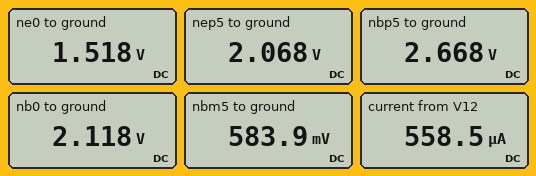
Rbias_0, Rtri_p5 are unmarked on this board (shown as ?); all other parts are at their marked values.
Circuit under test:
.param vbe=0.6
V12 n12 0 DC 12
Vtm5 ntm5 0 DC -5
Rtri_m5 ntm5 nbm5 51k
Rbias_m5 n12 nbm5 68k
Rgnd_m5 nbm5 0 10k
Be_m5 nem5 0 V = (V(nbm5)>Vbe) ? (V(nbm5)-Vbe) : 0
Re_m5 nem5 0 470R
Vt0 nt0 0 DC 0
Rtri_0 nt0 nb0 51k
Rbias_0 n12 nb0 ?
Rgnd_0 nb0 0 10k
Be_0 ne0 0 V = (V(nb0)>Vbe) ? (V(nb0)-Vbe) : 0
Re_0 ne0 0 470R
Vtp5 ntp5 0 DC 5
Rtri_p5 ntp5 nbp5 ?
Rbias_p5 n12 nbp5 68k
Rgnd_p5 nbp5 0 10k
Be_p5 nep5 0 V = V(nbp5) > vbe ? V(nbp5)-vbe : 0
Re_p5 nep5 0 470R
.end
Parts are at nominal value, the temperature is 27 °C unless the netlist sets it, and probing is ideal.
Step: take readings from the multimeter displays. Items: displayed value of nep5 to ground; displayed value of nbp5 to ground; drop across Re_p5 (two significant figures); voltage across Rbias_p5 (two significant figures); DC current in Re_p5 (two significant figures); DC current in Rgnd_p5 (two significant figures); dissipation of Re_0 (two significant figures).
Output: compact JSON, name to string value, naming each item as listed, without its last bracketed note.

{"displayed value of nep5 to ground": "2.068 V", "displayed value of nbp5 to ground": "2.668 V", "drop across Re_p5": "2.1 V", "voltage across Rbias_p5": "9.3 V", "DC current in Re_p5": "4.4 mA", "DC current in Rgnd_p5": "270 µA", "dissipation of Re_0": "4.9 mW"}
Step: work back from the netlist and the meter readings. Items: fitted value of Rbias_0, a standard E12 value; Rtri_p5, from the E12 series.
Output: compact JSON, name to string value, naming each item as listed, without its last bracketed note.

{"fitted value of Rbias_0, a standard E12 value": "39 kΩ", "Rtri_p5, from the E12 series": "18 kΩ"}
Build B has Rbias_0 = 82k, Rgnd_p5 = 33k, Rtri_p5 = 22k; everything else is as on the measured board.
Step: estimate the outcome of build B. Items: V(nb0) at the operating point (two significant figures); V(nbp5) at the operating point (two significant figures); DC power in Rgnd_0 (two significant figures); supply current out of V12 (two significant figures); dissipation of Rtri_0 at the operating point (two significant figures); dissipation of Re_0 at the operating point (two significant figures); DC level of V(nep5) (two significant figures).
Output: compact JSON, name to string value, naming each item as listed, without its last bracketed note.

{"V(nb0) at the operating point": "1.1 V", "V(nbp5) at the operating point": "4.5 V", "DC power in Rgnd_0": "120 µW", "supply current out of V12": "410 µA", "dissipation of Rtri_0 at the operating point": "24 µW", "dissipation of Re_0 at the operating point": "550 µW", "DC level of V(nep5)": "3.9 V"}
